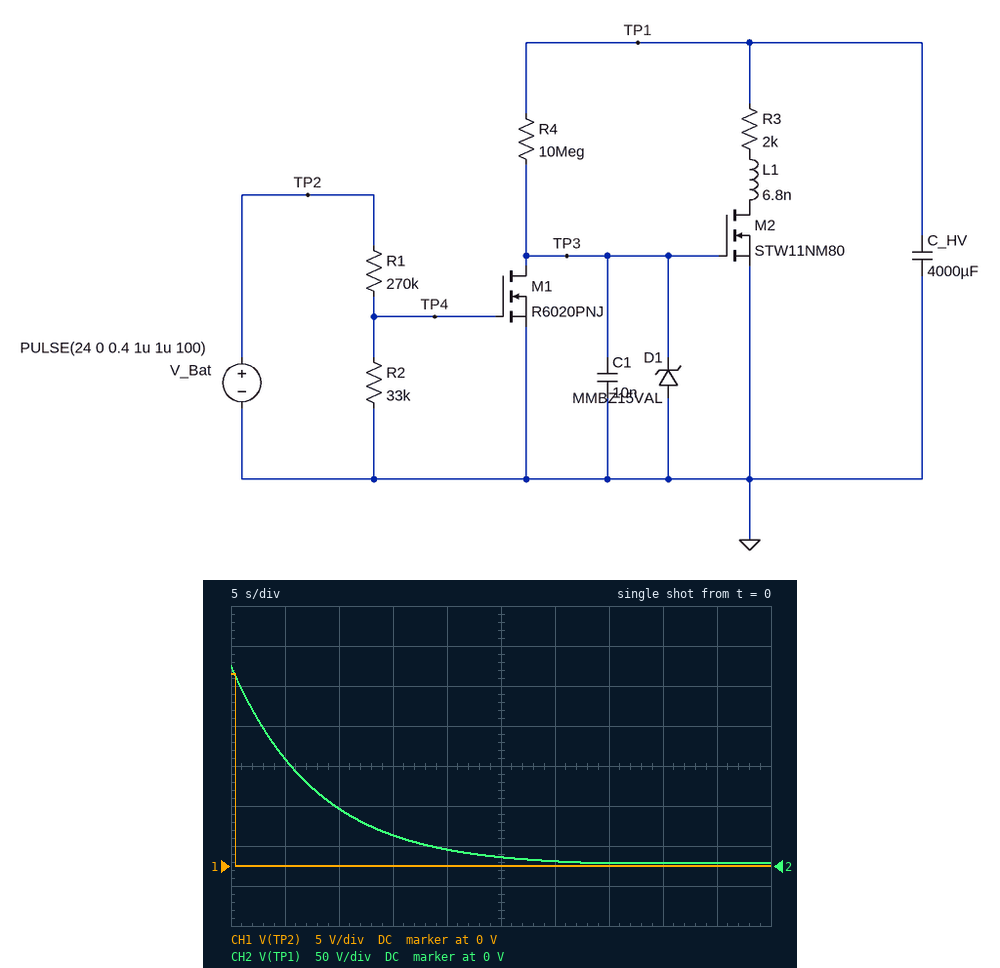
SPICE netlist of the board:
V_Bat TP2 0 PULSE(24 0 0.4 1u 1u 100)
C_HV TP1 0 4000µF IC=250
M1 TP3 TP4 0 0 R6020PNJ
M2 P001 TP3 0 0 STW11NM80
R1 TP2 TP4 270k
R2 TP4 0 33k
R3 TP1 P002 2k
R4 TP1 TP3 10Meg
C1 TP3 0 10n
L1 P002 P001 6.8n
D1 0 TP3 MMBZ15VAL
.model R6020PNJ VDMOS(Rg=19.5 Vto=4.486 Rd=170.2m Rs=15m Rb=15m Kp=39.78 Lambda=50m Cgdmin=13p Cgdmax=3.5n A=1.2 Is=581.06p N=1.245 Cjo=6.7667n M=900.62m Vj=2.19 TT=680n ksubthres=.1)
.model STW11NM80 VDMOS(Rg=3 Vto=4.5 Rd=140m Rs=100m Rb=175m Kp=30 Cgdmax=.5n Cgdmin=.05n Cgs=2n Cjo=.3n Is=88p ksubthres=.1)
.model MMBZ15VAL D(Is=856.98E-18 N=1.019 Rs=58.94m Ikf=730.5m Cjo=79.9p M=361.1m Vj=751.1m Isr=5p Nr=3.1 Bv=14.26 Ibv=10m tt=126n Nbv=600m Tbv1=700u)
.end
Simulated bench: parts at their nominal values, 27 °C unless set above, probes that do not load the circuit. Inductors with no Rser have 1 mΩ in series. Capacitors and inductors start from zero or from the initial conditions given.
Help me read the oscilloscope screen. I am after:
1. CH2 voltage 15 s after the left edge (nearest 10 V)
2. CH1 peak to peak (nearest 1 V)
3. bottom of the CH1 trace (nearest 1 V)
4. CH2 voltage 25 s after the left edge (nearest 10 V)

40 V
24 V
0 V
10 V
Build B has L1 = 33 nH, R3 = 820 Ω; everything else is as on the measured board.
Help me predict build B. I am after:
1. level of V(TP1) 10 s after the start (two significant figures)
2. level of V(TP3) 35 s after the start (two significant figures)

12 V
4.0 V
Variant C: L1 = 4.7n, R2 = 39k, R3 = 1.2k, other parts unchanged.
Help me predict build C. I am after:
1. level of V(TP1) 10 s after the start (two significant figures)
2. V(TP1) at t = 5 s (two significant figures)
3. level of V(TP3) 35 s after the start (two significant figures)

31 V
88 V
4.0 V
